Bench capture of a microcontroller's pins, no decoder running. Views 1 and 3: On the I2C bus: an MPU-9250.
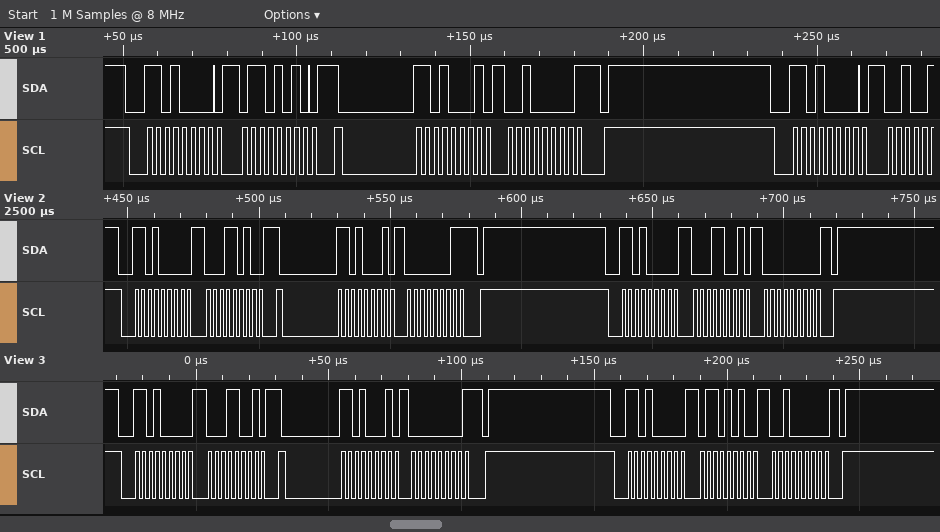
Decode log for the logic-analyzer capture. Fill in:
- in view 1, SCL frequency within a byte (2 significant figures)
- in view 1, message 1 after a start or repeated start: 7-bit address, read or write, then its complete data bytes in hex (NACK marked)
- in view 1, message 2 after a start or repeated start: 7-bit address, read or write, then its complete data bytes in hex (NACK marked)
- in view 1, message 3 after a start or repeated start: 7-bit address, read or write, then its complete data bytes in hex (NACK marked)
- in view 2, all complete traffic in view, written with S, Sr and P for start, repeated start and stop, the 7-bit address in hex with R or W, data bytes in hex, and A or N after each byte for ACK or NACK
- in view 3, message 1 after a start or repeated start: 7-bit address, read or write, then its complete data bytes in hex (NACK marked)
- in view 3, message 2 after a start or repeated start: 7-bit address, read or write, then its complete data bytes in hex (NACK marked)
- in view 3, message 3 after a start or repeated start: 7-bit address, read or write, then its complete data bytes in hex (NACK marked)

400 kHz
0x68 write: 6A
0x68 read: 20 NACK
0x68 write
S 68W A 1A A Sr 68R A 01 N P S 68W A 19 A 00 A P
0x68 write: 19
0x68 read: 00 NACK
0x68 write: 6A 20
